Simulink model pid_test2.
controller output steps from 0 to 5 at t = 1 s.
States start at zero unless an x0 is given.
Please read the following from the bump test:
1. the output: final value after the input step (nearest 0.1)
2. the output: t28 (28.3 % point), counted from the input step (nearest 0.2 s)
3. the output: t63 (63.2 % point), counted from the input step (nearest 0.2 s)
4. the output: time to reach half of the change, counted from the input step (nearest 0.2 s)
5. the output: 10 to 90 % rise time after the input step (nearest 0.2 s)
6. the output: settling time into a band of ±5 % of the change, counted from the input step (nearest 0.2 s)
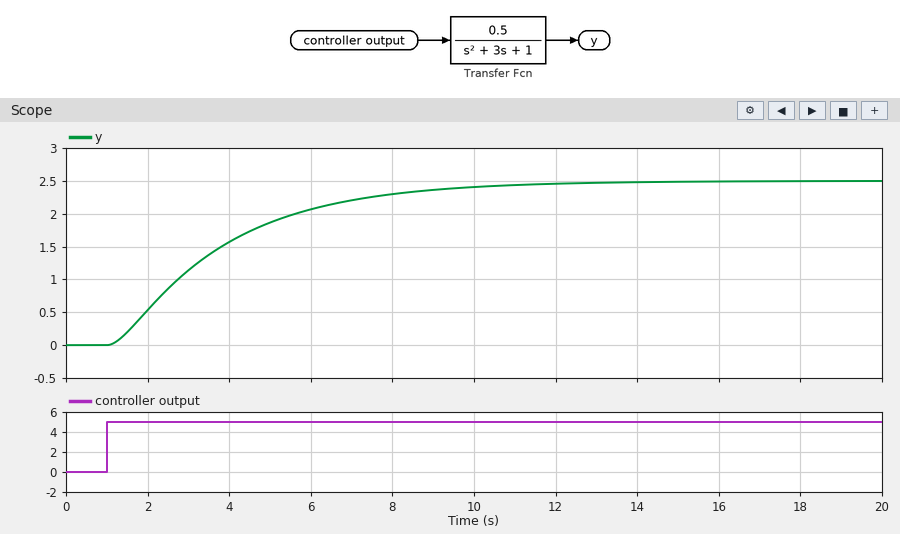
2.5
1.2 s
3.0 s
2.2 s
5.8 s
8.2 s
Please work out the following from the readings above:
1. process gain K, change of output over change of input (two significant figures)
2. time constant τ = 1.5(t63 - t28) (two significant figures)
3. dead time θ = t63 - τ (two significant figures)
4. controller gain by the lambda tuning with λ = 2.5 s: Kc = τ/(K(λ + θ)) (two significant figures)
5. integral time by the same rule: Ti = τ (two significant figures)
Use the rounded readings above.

0.50
2.7 s
0.30 s
1.9
2.7 s
